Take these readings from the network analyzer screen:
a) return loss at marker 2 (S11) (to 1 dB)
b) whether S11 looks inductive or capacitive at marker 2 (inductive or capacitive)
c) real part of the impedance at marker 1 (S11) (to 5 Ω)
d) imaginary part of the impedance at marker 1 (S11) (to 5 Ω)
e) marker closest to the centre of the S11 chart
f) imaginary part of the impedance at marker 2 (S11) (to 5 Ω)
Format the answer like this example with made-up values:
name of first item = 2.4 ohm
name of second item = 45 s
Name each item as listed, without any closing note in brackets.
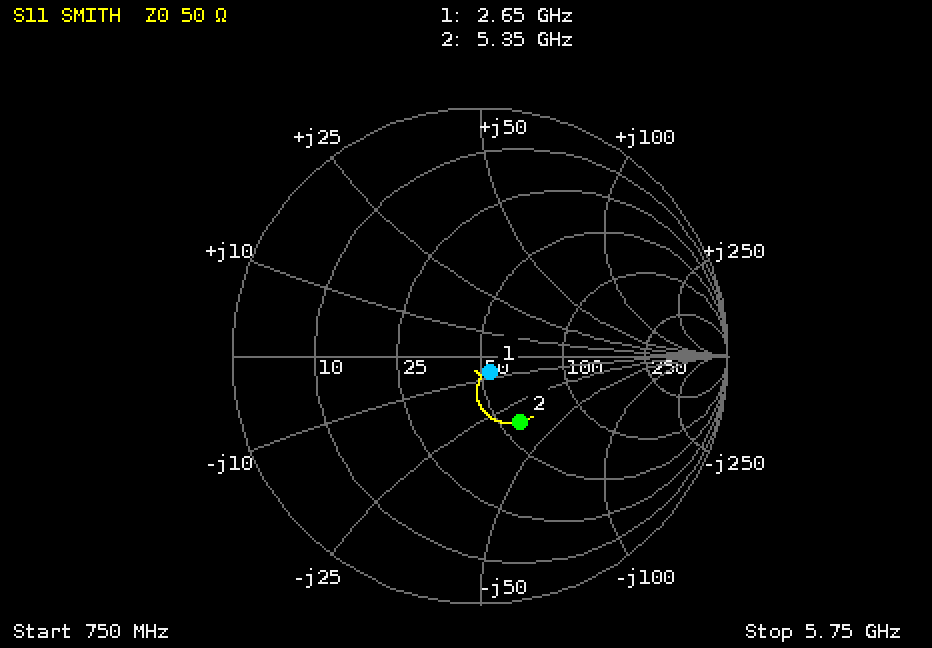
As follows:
return loss at marker 2 (S11) = 10 dB
whether S11 looks inductive or capacitive at marker 2 = capacitive
real part of the impedance at marker 1 (S11) = 55 Ω
imaginary part of the impedance at marker 1 (S11) = -5 Ω
marker closest to the centre of the S11 chart = marker 1
imaginary part of the impedance at marker 2 (S11) = -35 Ω
